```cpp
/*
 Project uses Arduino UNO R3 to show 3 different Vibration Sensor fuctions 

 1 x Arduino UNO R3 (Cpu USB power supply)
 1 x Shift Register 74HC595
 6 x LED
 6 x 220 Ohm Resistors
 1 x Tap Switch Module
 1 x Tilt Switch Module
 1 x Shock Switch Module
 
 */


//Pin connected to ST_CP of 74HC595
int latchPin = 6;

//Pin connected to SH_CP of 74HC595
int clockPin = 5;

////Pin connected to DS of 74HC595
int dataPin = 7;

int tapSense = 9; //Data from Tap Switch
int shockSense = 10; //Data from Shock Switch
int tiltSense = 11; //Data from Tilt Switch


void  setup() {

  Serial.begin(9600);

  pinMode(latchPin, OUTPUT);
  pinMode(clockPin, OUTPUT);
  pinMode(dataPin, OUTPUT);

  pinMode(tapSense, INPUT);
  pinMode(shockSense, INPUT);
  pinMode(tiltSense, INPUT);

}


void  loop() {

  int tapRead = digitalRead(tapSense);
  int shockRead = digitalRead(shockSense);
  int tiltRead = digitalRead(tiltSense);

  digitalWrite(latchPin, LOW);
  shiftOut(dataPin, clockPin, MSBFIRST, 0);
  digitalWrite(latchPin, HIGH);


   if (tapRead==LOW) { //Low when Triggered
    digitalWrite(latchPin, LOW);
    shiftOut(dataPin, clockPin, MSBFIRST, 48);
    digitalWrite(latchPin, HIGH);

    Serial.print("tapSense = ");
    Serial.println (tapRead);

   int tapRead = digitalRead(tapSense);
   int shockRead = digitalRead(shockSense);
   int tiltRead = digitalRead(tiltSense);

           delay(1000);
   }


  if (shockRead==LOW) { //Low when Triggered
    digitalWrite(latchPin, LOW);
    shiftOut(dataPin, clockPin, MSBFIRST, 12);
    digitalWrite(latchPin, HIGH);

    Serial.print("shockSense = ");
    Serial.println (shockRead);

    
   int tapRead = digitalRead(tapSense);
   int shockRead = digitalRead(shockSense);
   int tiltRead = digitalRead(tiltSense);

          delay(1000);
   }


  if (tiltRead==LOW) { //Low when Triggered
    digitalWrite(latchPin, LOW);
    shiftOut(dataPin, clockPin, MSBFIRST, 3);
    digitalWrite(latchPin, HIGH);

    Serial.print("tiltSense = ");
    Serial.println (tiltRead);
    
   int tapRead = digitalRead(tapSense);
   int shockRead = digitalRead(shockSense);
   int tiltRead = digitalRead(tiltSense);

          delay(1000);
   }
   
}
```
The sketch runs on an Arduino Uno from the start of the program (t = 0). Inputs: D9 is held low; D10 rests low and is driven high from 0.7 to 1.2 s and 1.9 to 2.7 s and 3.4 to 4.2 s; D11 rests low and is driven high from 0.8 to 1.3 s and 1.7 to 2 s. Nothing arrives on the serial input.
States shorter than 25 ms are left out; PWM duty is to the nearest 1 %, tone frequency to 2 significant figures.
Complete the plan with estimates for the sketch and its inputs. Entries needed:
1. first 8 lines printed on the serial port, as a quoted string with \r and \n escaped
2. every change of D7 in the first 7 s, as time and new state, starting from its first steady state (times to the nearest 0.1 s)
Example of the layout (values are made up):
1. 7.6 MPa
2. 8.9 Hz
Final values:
1. "tapSense = 0\r\nshockSense = 0\r\ntiltSense = 0\r\ntapSense = 0\r\nshockSense = 0\r\ntiltSense = 0\r\ntapSense = 0\r\nshockSense = 0\r\n"
2. 0 s low; 2 s high; 3 s low; 5 s high; 6 s low
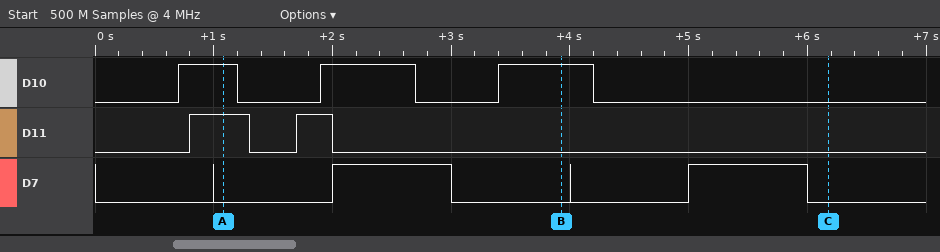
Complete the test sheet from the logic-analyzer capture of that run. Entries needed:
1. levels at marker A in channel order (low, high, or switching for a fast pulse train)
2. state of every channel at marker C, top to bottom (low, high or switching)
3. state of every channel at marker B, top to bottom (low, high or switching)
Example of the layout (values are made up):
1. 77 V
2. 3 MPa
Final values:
1. D10 high, D11 high, D7 low
2. D10 low, D11 low, D7 low
3. D10 high, D11 low, D7 low
